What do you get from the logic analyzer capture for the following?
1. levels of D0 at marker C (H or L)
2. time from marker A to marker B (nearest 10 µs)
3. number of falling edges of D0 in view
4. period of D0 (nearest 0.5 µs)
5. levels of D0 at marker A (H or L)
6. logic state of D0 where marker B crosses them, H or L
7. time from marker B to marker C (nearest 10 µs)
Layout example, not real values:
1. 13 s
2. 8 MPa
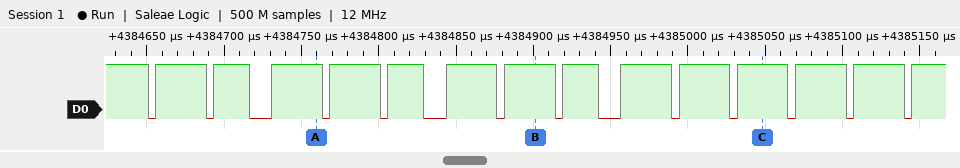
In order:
1. D0=H
2. 140 µs
3. 14
4. 37.5 µs
5. D0=H
6. D0=H
7. 150 µs
